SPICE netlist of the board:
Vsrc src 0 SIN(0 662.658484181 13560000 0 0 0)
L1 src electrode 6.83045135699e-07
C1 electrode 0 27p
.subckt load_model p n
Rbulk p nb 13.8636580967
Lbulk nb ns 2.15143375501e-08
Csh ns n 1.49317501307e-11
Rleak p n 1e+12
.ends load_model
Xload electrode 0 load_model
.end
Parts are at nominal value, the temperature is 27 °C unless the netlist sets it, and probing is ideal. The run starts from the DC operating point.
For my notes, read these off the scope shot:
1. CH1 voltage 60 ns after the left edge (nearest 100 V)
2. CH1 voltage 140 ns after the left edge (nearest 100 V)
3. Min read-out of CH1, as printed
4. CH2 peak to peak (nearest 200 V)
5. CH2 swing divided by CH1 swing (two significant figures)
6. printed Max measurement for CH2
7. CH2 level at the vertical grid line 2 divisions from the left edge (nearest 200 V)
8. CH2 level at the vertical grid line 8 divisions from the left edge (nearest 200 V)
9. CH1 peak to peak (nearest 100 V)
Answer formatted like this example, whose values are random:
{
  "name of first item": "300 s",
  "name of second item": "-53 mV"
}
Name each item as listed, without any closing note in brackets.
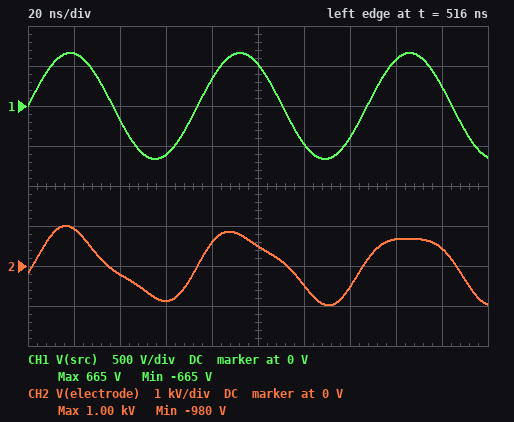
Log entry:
{
  "CH1 voltage 60 ns after the left edge": "-600 V",
  "CH1 voltage 140 ns after the left edge": "-400 V",
  "Min read-out of CH1, as printed": "-665 V",
  "CH2 peak to peak": "2.0 kV",
  "CH2 swing divided by CH1 swing": "1.5",
  "printed Max measurement for CH2": "1.00 kV",
  "CH2 level at the vertical grid line 2 divisions from the left edge": "-200 V",
  "CH2 level at the vertical grid line 8 divisions from the left edge": "600 V",
  "CH1 peak to peak": "1.3 kV"
}
